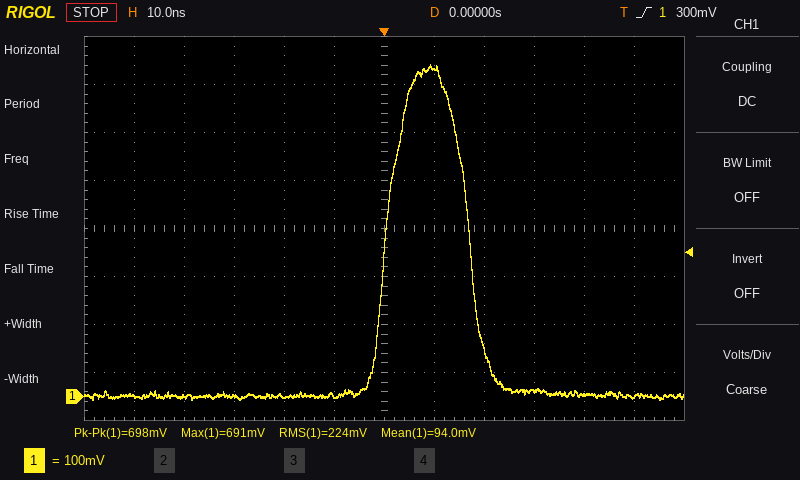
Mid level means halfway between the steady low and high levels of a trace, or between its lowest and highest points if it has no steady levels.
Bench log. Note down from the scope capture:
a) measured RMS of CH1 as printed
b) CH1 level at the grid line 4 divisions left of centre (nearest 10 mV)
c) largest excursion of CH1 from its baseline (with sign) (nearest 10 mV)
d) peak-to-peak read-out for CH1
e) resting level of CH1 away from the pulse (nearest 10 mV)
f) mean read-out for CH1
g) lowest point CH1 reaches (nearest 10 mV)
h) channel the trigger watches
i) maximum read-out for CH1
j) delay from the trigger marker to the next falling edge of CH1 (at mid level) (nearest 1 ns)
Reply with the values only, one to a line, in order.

224 mV
0 mV
+690 mV
698 mV
0 mV
94.0 mV
-10 mV
CH1
691 mV
17 ns
